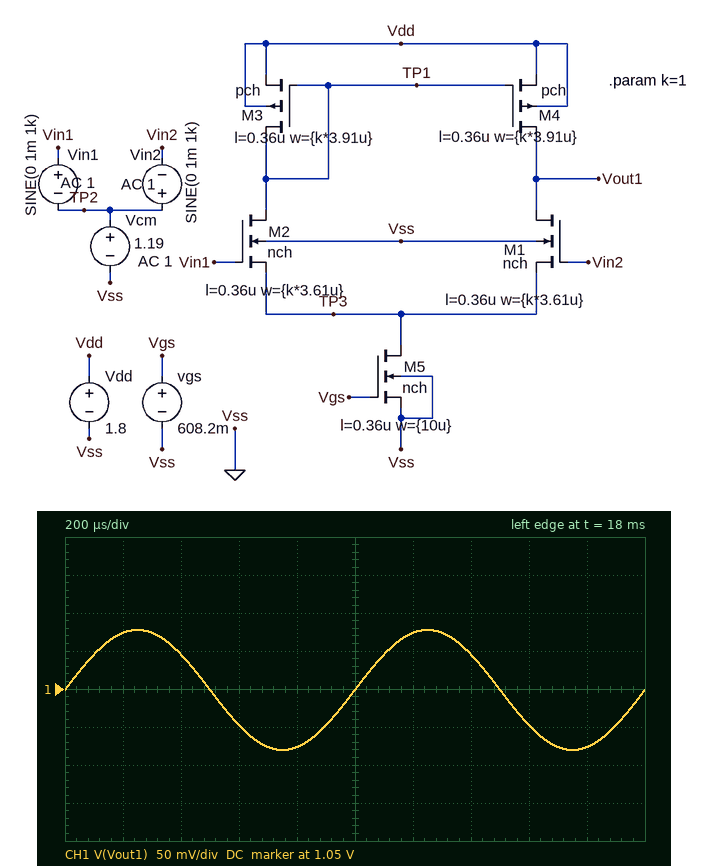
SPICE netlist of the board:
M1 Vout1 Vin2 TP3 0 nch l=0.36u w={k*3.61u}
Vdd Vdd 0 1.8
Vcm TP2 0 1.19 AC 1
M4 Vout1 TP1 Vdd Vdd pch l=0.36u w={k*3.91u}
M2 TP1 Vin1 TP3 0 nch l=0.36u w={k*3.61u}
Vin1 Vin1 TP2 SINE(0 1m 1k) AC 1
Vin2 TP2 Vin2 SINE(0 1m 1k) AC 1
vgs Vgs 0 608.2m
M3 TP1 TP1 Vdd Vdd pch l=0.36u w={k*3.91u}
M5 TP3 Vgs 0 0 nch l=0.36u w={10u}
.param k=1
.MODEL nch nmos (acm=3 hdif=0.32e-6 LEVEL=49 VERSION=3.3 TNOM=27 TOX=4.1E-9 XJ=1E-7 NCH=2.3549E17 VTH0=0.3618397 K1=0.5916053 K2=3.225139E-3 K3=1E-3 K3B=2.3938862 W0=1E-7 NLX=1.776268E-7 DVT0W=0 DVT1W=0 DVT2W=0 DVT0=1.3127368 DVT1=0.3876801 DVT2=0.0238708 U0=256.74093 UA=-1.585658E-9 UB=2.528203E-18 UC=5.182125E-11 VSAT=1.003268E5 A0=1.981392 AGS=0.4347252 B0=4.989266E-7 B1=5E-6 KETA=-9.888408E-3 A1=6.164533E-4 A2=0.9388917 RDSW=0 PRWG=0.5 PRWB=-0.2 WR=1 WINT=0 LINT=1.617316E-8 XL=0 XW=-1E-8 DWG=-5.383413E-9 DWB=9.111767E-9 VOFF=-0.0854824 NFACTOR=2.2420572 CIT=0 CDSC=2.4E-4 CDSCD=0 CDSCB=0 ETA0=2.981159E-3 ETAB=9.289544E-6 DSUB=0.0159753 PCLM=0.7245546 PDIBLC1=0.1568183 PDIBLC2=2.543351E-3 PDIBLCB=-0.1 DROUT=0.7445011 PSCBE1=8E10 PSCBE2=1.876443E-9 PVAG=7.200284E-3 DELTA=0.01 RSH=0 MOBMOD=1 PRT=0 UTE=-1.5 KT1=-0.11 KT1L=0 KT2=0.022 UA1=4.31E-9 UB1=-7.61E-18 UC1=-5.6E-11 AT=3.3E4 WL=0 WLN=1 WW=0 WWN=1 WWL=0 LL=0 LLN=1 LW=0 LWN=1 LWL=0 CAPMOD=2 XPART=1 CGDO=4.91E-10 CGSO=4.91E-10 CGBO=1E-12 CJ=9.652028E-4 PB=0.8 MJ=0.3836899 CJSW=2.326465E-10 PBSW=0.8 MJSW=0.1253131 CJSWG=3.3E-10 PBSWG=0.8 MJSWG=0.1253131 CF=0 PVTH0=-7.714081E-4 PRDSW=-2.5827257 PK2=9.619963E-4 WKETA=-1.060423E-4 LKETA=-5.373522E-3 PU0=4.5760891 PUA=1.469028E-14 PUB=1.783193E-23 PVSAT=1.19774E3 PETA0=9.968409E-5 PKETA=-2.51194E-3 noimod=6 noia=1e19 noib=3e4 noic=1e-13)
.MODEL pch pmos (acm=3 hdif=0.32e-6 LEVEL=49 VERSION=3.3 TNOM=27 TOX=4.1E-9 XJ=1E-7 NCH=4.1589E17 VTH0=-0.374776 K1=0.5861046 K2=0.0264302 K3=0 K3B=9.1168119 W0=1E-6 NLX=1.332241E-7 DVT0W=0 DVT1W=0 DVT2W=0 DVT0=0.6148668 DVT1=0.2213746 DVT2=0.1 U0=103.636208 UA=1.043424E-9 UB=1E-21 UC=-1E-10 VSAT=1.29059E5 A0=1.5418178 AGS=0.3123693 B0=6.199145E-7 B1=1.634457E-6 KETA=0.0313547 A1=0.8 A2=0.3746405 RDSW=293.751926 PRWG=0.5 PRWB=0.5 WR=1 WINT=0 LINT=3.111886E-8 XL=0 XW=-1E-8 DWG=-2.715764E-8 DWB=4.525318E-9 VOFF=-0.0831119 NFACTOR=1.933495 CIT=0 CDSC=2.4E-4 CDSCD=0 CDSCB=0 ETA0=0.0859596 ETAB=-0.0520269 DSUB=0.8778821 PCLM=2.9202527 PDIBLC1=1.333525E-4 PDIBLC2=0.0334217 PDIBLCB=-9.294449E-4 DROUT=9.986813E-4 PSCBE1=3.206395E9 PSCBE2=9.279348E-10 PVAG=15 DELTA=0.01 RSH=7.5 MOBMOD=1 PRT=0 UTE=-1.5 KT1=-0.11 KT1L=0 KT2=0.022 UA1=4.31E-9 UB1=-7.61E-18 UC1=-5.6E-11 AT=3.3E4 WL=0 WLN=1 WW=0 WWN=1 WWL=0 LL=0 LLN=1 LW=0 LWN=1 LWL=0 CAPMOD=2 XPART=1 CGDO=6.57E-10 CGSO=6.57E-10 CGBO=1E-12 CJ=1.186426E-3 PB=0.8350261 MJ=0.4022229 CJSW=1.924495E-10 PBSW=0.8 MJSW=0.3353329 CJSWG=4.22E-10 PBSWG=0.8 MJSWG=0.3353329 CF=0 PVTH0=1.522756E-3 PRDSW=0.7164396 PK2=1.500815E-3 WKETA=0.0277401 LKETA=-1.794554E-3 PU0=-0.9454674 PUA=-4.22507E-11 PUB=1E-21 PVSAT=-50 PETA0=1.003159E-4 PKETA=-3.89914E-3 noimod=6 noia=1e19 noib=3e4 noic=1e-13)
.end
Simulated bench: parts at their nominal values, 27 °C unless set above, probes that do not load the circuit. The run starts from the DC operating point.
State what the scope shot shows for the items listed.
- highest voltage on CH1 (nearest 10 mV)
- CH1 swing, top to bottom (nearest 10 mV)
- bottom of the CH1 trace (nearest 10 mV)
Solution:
1.13 V
160 mV
970 mV
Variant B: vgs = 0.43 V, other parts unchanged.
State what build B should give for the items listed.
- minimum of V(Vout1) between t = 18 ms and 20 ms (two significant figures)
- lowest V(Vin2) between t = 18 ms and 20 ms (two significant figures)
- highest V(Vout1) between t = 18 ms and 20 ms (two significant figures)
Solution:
1.2 V
1.2 V
1.4 V
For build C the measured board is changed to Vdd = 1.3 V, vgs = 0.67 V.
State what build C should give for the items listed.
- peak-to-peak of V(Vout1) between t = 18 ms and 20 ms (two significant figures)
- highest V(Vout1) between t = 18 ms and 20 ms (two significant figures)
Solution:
1.9 mV
410 mV
